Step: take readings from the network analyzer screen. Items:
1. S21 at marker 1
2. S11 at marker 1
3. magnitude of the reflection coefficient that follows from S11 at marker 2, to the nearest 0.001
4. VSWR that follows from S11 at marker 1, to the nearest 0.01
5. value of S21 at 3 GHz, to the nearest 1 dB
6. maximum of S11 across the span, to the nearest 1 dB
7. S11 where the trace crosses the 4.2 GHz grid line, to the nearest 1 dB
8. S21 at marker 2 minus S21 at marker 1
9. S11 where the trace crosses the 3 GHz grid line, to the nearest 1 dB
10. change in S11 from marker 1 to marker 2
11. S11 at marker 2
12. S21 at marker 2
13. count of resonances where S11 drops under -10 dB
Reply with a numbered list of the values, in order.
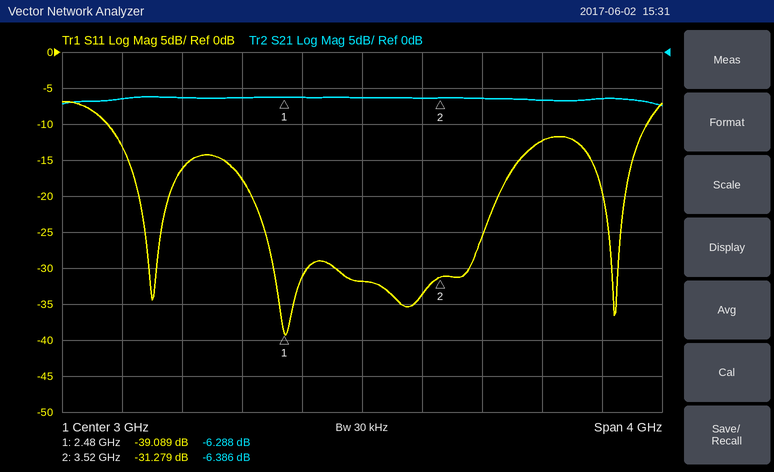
1. -6.288 dB
2. -39.089 dB
3. 0.027
4. 1.02
5. -6 dB
6. -7 dB
7. -12 dB
8. -0.098 dB
9. -32 dB
10. 7.810 dB
11. -31.279 dB
12. -6.386 dB
13. 4
